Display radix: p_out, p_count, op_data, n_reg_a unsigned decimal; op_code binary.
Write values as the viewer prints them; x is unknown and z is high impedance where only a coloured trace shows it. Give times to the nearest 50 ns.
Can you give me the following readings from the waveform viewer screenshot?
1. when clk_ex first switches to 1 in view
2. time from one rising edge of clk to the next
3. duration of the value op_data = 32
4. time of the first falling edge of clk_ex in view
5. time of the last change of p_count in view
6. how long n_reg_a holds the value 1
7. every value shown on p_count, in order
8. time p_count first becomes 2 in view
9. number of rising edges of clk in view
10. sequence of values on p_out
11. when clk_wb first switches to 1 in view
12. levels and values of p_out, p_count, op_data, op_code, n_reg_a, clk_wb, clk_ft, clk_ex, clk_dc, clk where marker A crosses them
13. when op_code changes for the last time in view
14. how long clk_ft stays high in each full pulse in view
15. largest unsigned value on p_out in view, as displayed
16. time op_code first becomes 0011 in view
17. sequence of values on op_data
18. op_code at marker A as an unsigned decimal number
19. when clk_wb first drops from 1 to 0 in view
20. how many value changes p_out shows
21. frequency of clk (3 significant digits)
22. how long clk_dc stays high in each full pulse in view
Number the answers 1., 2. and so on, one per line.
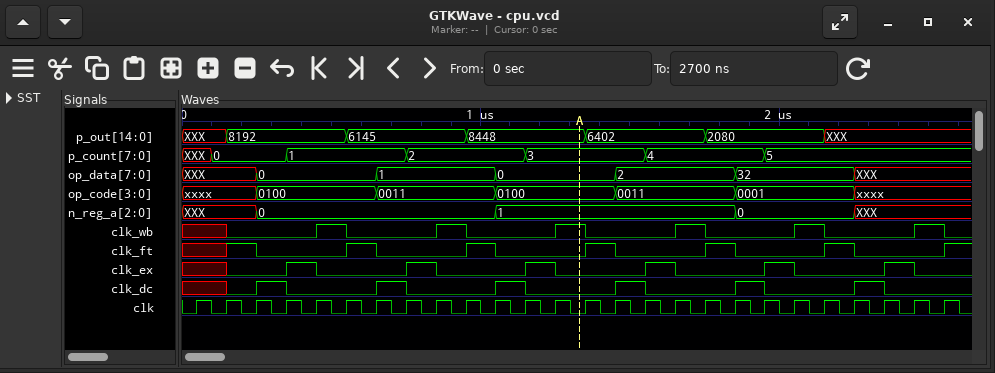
1. 350 ns
2. 100 ns
3. 400 ns
4. 450 ns
5. 1950 ns
6. 800 ns
7. XXX, 0, 1, 2, 3, 4, 5
8. 750 ns
9. 26
10. XXX, 8192, 6145, 8448, 6402, 2080, XXX
11. 450 ns
12. p_out=8448, p_count=3, op_data=0, op_code=0100, n_reg_a=1, clk_wb=1, clk_ft=0, clk_ex=0, clk_dc=0, clk=0
13. 2250 ns
14. 100 ns, 100 ns, 100 ns, 100 ns, 100 ns
15. 8448
16. 650 ns
17. XXX, 0, 1, 0, 2, 32, XXX
18. 4
19. 550 ns
20. 6
21. 10.0 MHz
22. 100 ns, 100 ns, 100 ns, 100 ns, 100 ns, 100 ns
